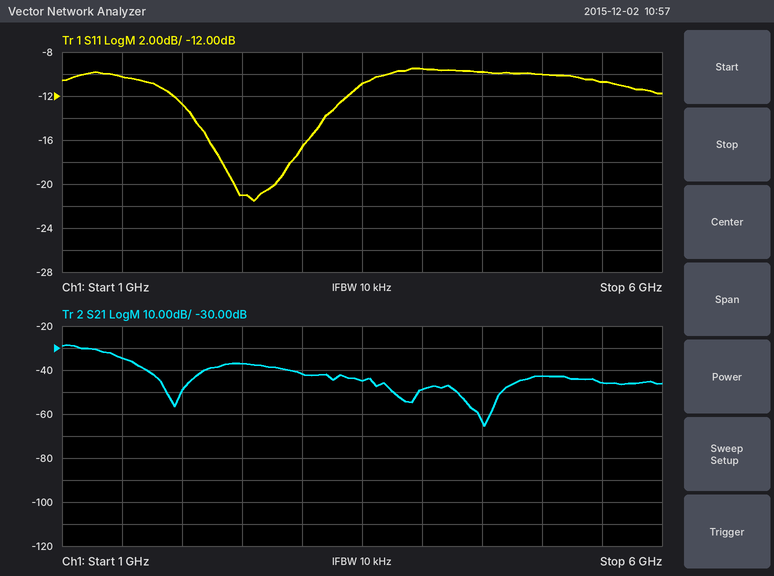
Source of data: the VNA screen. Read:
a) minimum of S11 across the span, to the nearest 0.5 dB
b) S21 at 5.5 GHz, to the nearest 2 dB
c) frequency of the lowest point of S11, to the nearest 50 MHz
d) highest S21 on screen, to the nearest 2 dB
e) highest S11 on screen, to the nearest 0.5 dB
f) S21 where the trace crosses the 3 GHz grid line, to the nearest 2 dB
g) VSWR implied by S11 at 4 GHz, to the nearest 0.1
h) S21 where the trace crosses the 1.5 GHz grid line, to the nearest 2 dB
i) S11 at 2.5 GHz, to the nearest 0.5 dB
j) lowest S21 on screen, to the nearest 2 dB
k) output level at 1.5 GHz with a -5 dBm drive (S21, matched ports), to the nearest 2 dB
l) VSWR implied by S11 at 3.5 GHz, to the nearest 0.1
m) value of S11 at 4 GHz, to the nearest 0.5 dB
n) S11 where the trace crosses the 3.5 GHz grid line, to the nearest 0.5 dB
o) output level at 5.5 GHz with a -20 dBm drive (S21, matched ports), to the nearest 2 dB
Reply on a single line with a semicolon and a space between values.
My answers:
-21.5 dB; -46 dB; 2.60 GHz; -28 dB; -9.5 dB; -42 dB; 2.0; -34 dB; -21.0 dB; -66 dB; -40 dBm; 1.8; -9.5 dB; -11.0 dB; -66 dBm
